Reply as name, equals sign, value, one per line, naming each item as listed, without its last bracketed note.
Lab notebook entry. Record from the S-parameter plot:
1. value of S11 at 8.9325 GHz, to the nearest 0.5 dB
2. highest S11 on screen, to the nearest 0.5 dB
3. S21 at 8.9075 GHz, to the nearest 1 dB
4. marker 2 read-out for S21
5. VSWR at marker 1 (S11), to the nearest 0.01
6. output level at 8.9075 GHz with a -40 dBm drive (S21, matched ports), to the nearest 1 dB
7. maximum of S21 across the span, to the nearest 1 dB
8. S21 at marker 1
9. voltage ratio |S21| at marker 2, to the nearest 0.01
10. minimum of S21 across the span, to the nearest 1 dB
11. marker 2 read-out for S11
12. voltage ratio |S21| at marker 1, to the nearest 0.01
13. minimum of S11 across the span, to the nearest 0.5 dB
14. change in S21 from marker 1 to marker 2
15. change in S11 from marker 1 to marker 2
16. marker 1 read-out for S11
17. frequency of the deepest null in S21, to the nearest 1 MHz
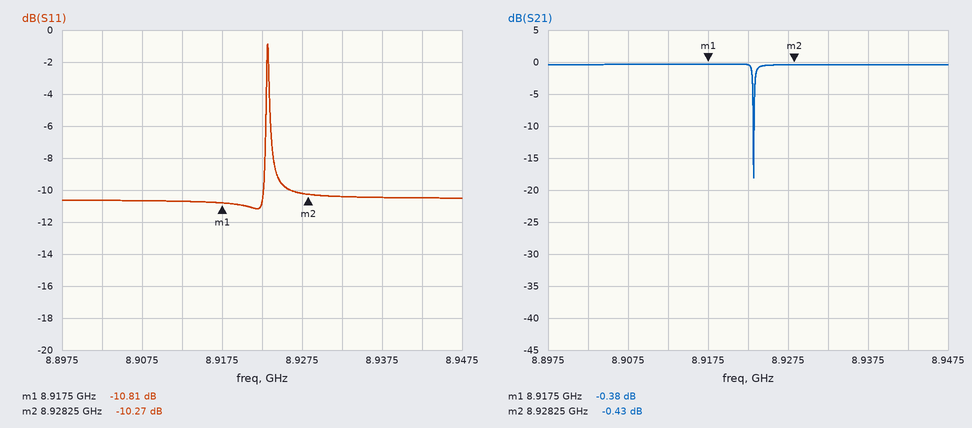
value of S11 at 8.9325 GHz, to the nearest 0.5 dB = -10.5 dB
highest S11 on screen, to the nearest 0.5 dB = -1.0 dB
S21 at 8.9075 GHz, to the nearest 1 dB = 0 dB
marker 2 read-out for S21 = -0.43 dB
VSWR at marker 1 (S11), to the nearest 0.01 = 1.81
output level at 8.9075 GHz with a -40 dBm drive (S21, matched ports), to the nearest 1 dB = -40 dBm
maximum of S21 across the span, to the nearest 1 dB = 0 dB
S21 at marker 1 = -0.38 dB
voltage ratio |S21| at marker 2, to the nearest 0.01 = 0.95
minimum of S21 across the span, to the nearest 1 dB = -18 dB
marker 2 read-out for S11 = -10.27 dB
voltage ratio |S21| at marker 1, to the nearest 0.01 = 0.96
minimum of S11 across the span, to the nearest 0.5 dB = -11.0 dB
change in S21 from marker 1 to marker 2 = -0.05 dB
change in S11 from marker 1 to marker 2 = 0.54 dB
marker 1 read-out for S11 = -10.81 dB
frequency of the deepest null in S21, to the nearest 1 MHz = 8.923 GHz
